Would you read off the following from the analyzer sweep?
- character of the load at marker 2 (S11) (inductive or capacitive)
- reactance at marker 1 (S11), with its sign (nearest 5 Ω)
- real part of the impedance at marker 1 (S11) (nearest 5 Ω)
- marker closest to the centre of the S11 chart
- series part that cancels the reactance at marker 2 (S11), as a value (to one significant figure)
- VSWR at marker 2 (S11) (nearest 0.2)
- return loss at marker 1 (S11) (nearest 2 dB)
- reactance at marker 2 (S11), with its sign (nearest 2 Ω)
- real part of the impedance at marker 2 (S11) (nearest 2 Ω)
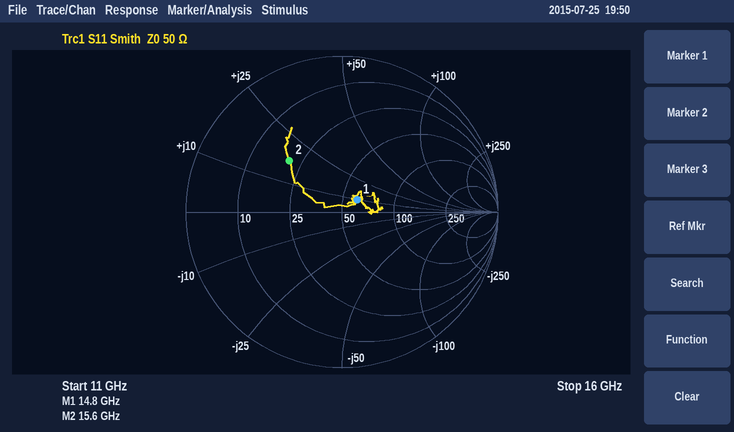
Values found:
inductive
+10 Ω
60 Ω
marker 1
600 fF
2.8
18 dB
+18 Ω
20 Ω
